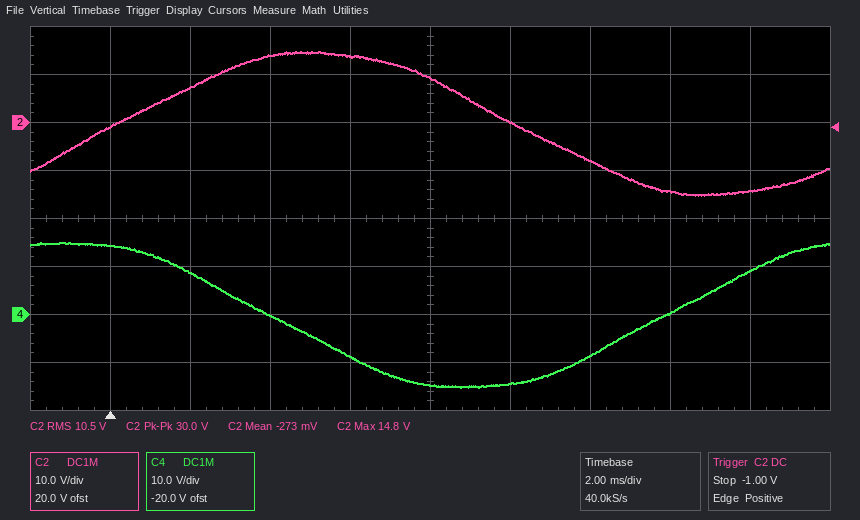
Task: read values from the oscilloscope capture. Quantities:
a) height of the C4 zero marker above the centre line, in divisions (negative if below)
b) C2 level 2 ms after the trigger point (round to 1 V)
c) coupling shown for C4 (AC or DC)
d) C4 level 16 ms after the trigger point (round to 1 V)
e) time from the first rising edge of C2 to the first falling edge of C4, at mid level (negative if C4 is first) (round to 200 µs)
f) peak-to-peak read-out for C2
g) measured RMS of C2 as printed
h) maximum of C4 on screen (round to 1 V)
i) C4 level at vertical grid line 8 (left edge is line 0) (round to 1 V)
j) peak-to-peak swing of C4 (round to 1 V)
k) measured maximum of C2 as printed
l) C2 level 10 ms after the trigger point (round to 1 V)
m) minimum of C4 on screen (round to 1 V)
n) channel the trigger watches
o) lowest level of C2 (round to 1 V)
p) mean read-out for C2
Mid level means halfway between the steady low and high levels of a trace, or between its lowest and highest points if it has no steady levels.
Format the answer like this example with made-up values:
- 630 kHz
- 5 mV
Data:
- -2.0 div
- 7 V
- DC
- 9 V
- +3.8 ms
- 30.0 V
- 10.5 V
- 15 V
- 0 V
- 30 V
- 14.8 V
- 0 V
- -15 V
- C2
- -15 V
- -273 mV
